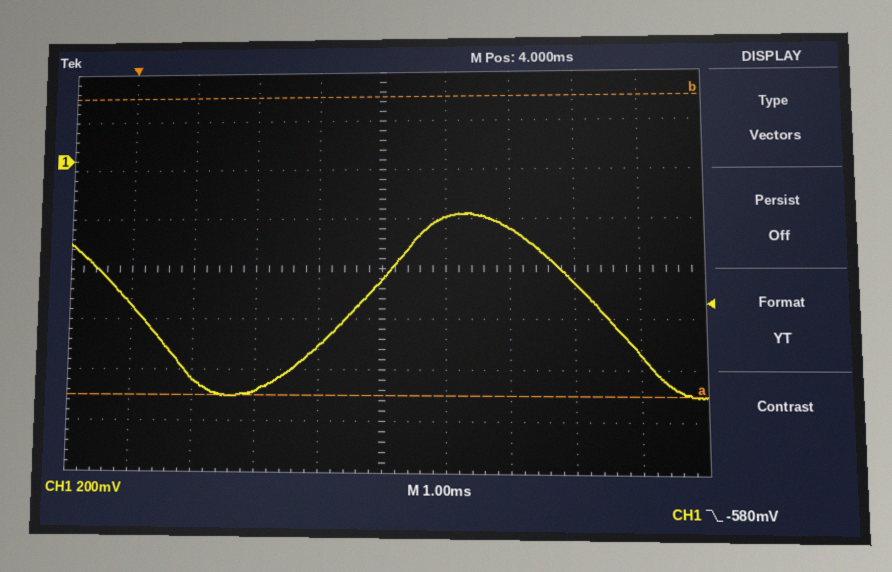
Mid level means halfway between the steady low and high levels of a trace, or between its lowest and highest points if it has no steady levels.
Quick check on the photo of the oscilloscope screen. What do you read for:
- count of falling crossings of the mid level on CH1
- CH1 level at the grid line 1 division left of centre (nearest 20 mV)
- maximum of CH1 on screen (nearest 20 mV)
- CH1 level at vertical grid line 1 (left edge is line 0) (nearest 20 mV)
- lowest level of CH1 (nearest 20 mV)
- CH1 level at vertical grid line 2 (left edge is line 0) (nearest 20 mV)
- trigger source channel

2
-740 mV
-220 mV
-580 mV
-940 mV
-880 mV
CH1
